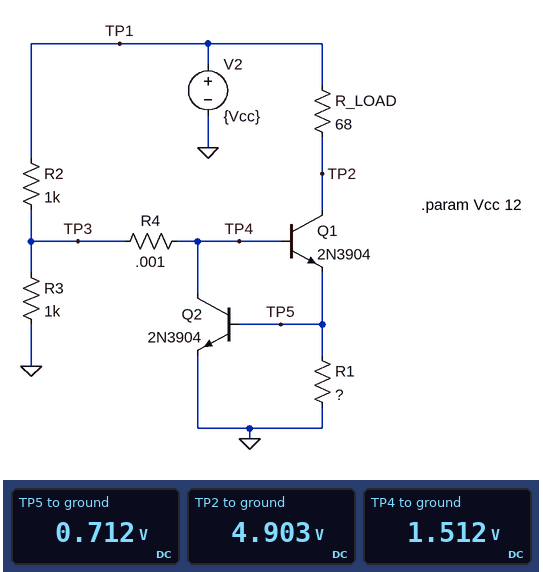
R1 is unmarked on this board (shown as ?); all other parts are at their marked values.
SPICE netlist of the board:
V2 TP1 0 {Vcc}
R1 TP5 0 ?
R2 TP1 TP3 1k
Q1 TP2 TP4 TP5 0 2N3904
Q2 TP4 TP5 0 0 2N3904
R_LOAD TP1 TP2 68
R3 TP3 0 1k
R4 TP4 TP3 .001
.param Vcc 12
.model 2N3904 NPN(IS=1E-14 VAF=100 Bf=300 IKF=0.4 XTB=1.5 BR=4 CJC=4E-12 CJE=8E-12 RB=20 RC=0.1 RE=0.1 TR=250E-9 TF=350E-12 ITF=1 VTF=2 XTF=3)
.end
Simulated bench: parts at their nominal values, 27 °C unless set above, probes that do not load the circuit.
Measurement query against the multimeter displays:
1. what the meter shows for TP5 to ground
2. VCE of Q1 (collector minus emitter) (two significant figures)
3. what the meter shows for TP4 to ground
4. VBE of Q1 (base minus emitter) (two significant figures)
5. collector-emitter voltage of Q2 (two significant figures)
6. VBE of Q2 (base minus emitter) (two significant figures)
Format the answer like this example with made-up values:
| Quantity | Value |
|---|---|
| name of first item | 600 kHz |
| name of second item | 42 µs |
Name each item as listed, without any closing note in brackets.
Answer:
| Quantity | Value |
|---|---|
| what the meter shows for TP5 to ground | 0.712 V |
| VCE of Q1 (collector minus emitter) | 4.2 V |
| what the meter shows for TP4 to ground | 1.512 V |
| VBE of Q1 (base minus emitter) | 800 mV |
| collector-emitter voltage of Q2 | 1.5 V |
| VBE of Q2 (base minus emitter) | 710 mV |
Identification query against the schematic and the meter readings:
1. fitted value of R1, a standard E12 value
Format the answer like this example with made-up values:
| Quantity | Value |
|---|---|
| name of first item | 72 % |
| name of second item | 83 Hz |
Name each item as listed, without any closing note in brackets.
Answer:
| Quantity | Value |
|---|---|
| fitted value of R1, a standard E12 value | 6.8 Ω |
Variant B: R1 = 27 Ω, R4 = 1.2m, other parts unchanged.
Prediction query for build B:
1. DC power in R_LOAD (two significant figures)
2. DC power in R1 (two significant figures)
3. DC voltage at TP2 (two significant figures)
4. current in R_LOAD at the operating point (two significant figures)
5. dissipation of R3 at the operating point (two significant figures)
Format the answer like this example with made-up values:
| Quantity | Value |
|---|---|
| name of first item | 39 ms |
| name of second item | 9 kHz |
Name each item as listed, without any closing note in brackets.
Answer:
| Quantity | Value |
|---|---|
| DC power in R_LOAD | 47 mW |
| DC power in R1 | 19 mW |
| DC voltage at TP2 | 10 V |
| current in R_LOAD at the operating point | 26 mA |
| dissipation of R3 at the operating point | 2.1 mW |
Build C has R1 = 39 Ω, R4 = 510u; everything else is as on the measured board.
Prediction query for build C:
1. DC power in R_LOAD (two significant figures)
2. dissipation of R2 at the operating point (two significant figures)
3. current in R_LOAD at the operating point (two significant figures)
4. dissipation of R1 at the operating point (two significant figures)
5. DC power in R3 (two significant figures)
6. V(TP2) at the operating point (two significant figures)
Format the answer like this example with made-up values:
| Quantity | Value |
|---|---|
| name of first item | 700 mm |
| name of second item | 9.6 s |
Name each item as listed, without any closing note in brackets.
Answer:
| Quantity | Value |
|---|---|
| DC power in R_LOAD | 23 mW |
| dissipation of R2 at the operating point | 110 mW |
| current in R_LOAD at the operating point | 18 mA |
| dissipation of R1 at the operating point | 13 mW |
| DC power in R3 | 2.1 mW |
| V(TP2) at the operating point | 11 V |
